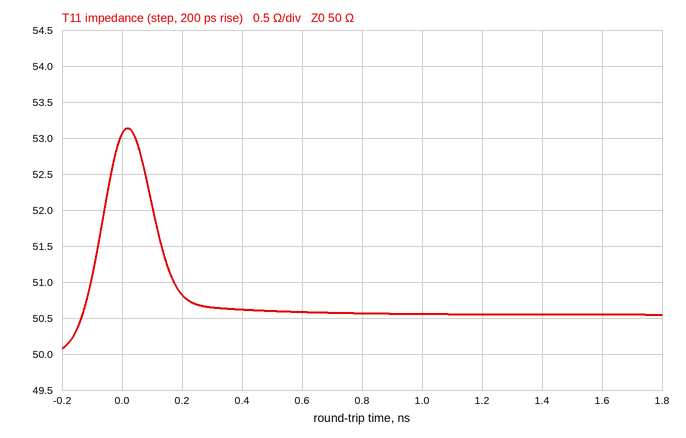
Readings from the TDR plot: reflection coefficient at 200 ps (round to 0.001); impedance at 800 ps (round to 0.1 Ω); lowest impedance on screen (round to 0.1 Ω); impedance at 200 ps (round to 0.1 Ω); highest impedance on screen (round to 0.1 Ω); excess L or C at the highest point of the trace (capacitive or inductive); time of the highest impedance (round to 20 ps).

+0.008
50.6 Ω
50.1 Ω
50.8 Ω
53.1 Ω
inductive
20 ps
